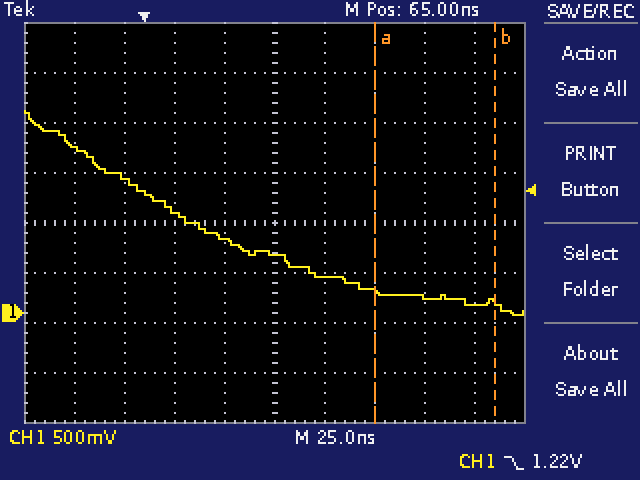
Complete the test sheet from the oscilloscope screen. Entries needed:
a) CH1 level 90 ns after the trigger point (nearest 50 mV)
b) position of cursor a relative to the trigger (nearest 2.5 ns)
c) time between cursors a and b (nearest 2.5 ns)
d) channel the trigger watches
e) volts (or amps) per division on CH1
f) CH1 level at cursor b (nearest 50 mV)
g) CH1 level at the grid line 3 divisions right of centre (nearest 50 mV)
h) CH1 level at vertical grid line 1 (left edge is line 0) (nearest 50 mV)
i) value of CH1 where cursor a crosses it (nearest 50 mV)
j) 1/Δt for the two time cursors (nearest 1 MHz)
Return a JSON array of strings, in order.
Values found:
["350 mV", "+115.0 ns", "60.0 ns", "CH1", "500 mV", "100 mV", "150 mV", "1.65 V", "200 mV", "17 MHz"]
